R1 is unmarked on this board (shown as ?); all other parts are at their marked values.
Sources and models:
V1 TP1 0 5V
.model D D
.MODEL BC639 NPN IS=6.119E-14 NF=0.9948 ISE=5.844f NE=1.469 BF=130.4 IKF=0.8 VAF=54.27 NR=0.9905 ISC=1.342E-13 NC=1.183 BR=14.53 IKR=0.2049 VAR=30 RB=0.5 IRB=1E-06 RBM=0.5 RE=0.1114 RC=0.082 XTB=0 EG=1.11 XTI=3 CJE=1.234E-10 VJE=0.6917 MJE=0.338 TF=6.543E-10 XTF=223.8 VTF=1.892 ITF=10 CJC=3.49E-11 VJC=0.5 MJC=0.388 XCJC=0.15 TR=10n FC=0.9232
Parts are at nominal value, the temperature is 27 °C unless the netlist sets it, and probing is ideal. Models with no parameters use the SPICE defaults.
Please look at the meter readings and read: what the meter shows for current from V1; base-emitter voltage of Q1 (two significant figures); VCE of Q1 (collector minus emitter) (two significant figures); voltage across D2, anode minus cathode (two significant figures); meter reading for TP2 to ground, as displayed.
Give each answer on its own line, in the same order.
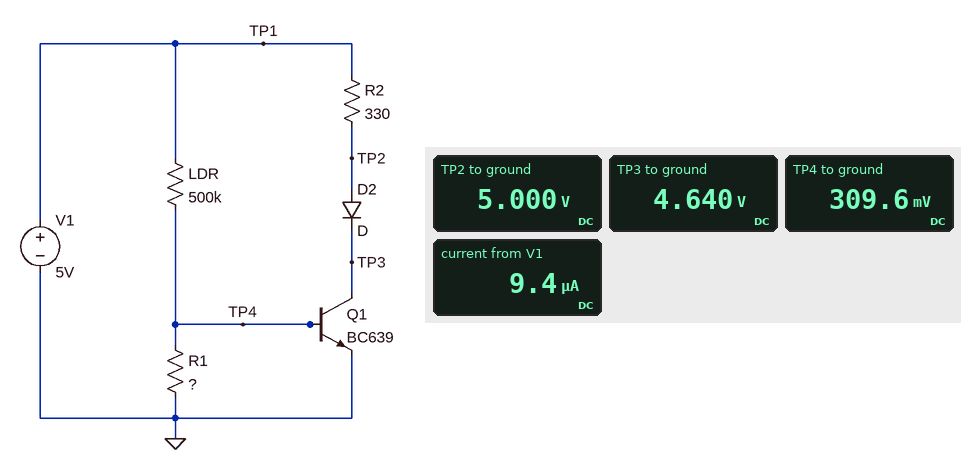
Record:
9.4 µA
310 mV
4.6 V
360 mV
5.000 V
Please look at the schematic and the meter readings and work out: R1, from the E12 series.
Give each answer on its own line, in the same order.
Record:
33 kΩ
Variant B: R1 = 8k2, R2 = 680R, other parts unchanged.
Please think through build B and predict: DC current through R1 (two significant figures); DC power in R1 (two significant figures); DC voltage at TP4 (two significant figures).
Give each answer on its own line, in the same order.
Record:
9.8 µA
790 nW
81 mV
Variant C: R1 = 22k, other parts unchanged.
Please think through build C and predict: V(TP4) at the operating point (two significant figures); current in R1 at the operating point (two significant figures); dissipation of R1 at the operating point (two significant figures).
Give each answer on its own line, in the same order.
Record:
210 mV
9.6 µA
2.0 µW
